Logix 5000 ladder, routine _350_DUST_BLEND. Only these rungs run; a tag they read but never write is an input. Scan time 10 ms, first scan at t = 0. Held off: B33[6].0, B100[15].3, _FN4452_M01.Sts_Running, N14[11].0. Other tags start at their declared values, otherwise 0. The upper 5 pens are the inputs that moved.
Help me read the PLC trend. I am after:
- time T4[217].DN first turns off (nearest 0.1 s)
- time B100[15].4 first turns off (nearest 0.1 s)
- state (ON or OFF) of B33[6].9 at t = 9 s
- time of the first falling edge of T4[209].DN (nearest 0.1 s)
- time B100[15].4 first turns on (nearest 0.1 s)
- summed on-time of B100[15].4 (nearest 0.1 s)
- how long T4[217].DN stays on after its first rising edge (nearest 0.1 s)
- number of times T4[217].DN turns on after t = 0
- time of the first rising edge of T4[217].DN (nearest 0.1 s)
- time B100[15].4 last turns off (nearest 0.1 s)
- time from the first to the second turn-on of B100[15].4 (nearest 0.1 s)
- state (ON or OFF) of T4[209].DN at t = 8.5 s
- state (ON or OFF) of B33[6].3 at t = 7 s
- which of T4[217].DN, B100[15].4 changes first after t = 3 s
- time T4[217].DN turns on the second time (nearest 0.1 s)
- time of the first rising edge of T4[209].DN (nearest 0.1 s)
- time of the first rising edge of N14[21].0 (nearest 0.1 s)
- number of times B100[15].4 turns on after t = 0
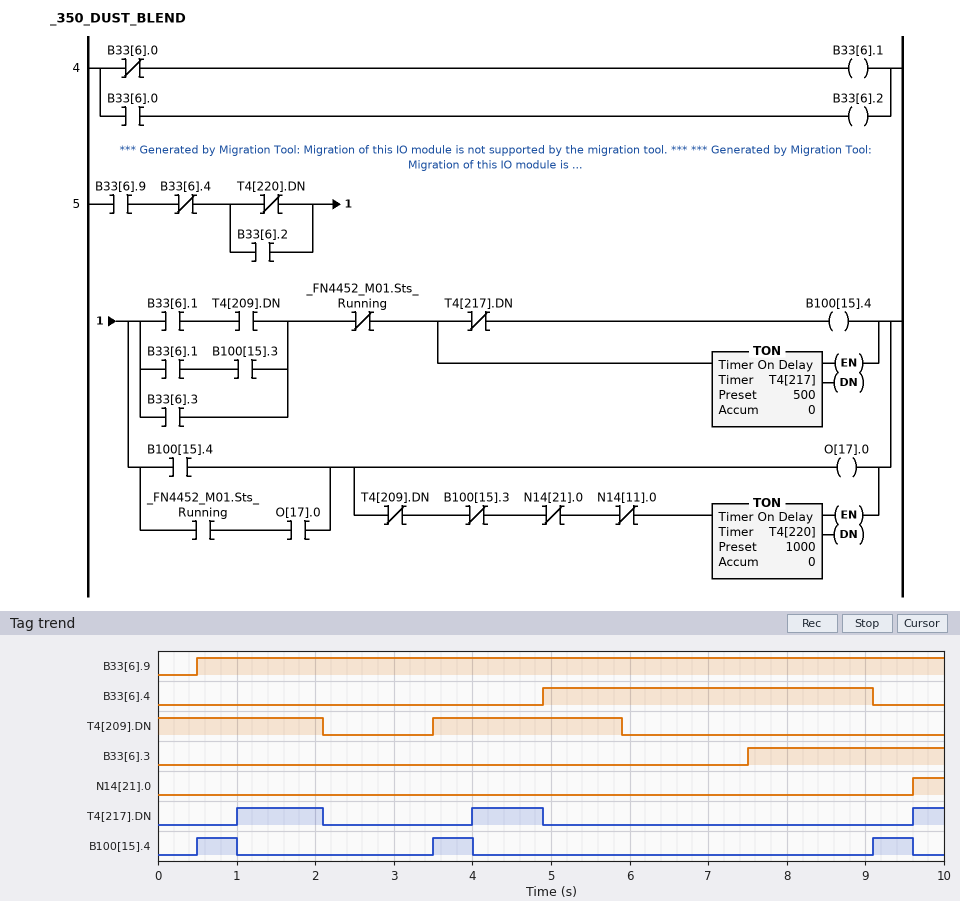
2.1 s
1.0 s
ON
2.1 s
0.5 s
1.5 s
1.1 s
3
1.0 s
9.6 s
3.0 s
OFF
OFF
B100[15].4
4.0 s
3.5 s
9.6 s
3
